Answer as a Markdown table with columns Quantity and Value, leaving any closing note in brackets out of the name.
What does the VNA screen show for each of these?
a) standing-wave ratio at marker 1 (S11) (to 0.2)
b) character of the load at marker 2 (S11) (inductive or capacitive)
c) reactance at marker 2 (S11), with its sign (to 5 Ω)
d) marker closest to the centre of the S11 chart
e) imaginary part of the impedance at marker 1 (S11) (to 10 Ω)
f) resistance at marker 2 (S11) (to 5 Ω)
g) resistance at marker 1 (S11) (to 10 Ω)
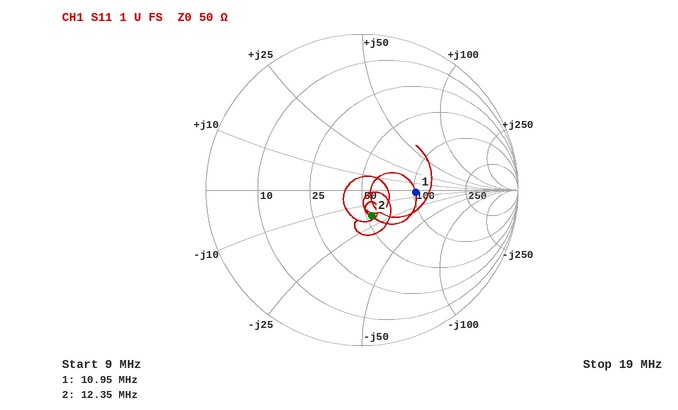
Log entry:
| Quantity | Value |
|---|---|
| standing-wave ratio at marker 1 (S11) | 2.0 |
| character of the load at marker 2 (S11) | capacitive |
| reactance at marker 2 (S11), with its sign | -20 Ω |
| marker closest to the centre of the S11 chart | marker 2 |
| imaginary part of the impedance at marker 1 (S11) | 0 Ω |
| resistance at marker 2 (S11) | 55 Ω |
| resistance at marker 1 (S11) | 100 Ω |
